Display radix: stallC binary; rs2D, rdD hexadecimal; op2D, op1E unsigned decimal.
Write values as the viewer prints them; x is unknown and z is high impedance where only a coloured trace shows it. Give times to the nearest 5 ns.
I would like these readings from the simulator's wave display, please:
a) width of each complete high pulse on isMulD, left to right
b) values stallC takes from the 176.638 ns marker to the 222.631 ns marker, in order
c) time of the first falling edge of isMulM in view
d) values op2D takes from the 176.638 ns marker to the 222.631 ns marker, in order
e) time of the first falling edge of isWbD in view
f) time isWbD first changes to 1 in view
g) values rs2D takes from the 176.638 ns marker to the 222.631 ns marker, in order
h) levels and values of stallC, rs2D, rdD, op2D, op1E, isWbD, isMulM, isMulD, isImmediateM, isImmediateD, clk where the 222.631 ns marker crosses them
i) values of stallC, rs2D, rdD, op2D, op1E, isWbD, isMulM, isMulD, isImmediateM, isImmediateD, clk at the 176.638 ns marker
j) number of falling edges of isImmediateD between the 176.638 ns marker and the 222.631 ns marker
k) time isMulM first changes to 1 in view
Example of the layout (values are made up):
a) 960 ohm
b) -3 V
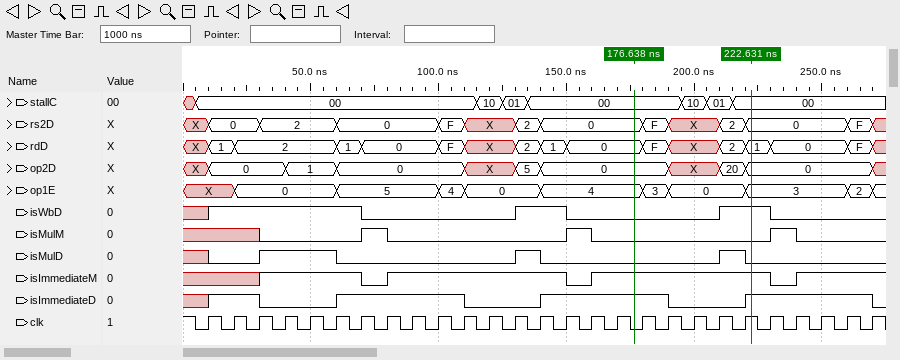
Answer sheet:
a) 30 ns, 10 ns, 10 ns
b) 00, 10, 01, 00
c) 80 ns
d) 0, X, 20, 0
e) 70 ns
f) 10 ns
g) 0, F, X, 2, 0
h) stallC=00, rs2D=0, rdD=1, op2D=0, op1E=3, isWbD=1, isMulM=0, isMulD=0, isImmediateM=1, isImmediateD=1, clk=1
i) stallC=00, rs2D=0, rdD=0, op2D=0, op1E=4, isWbD=0, isMulM=0, isMulD=0, isImmediateM=1, isImmediateD=1, clk=0
j) 1
k) 70 ns
